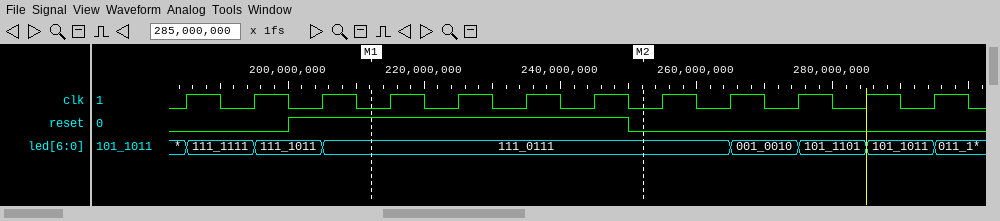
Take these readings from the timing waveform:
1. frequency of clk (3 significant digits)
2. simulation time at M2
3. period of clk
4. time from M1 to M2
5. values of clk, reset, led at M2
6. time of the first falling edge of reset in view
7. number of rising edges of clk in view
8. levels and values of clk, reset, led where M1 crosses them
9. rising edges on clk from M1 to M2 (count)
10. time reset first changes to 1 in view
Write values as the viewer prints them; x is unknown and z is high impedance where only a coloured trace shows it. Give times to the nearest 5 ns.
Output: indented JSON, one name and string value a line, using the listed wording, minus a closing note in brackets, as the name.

{
  "frequency of clk": "100 MHz",
  "simulation time at M2": "250 ns",
  "period of clk": "10 ns",
  "time from M1 to M2": "40 ns",
  "values of clk, reset, led at M2": "clk=0, reset=0, led=111_0111",
  "time of the first falling edge of reset in view": "250 ns",
  "number of rising edges of clk in view": "12",
  "levels and values of clk, reset, led where M1 crosses them": "clk=0, reset=1, led=111_0111",
  "rising edges on clk from M1 to M2": "4",
  "time reset first changes to 1 in view": "200 ns"
}
